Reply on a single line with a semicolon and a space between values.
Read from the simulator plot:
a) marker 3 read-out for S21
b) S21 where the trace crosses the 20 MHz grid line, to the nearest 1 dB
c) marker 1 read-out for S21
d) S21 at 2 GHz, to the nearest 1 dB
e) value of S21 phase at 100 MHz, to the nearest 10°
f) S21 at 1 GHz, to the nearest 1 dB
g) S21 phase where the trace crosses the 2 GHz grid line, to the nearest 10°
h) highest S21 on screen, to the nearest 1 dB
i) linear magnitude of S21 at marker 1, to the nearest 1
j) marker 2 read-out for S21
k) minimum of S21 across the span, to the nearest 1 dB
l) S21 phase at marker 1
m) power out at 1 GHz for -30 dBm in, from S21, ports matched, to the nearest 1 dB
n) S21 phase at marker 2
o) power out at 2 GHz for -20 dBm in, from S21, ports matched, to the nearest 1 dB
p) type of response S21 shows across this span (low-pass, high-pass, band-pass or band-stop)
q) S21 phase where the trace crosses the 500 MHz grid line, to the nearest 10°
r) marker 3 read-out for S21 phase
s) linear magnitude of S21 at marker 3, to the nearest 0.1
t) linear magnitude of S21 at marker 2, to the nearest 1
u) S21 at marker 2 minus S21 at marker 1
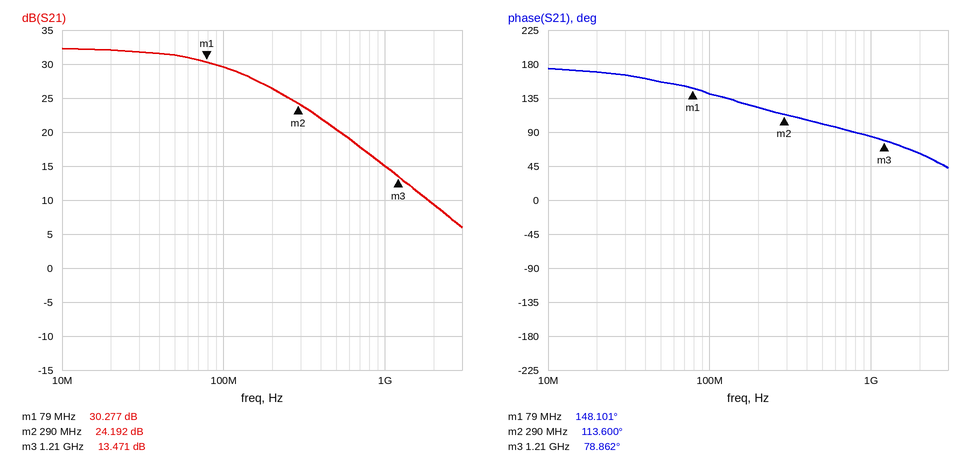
13.471 dB; 32 dB; 30.277 dB; 9 dB; 140°; 15 dB; 60°; 32 dB; 33; 24.192 dB; 6 dB; 148.101°; -15 dBm; 113.600°; -11 dBm; low-pass; 100°; 78.862°; 4.7; 16; -6.085 dB
